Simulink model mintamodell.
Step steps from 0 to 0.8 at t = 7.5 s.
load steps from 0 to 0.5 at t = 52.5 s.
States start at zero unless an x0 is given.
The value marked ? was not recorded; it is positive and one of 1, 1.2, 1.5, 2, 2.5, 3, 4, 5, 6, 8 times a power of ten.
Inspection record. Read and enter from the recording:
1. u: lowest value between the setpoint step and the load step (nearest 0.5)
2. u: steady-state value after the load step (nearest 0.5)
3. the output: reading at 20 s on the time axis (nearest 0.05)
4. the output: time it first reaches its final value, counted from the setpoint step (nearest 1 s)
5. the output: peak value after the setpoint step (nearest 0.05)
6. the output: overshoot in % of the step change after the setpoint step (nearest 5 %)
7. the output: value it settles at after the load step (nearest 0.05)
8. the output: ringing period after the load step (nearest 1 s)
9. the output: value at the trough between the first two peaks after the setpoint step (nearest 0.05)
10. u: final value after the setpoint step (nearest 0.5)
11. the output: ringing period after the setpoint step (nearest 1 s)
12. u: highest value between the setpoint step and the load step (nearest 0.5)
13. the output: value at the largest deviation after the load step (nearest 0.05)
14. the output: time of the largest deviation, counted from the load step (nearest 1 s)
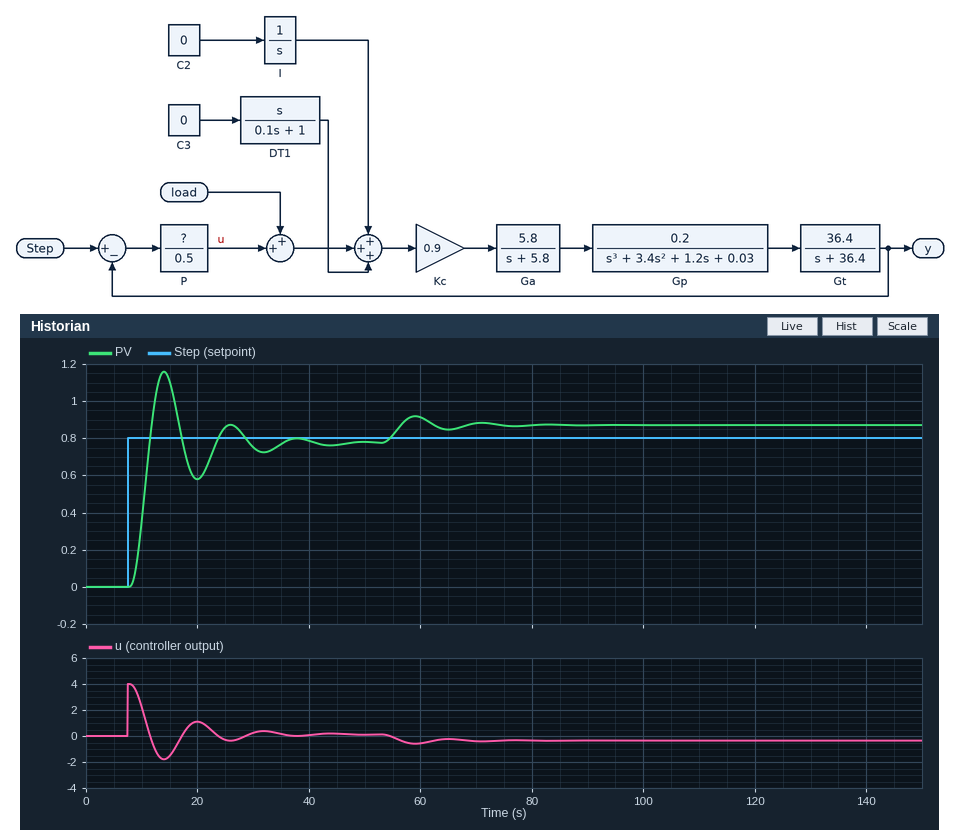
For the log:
-2.0
-0.5
0.60
4 s
1.15
50 %
0.85
12 s
0.60
0.0
12 s
4.0
0.90
7 s
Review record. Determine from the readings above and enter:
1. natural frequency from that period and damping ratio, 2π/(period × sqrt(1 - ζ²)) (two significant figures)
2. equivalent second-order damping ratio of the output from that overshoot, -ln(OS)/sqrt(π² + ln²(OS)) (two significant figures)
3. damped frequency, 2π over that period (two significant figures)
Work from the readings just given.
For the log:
0.54 rad/s
0.22
0.52 rad/s
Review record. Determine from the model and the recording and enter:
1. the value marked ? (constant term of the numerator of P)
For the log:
2.5
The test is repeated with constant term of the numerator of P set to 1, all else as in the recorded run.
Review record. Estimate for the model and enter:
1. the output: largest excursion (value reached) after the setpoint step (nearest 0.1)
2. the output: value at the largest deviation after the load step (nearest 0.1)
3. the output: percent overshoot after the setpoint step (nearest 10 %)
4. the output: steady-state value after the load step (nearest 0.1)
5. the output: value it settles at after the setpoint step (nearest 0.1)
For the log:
0.9
1.0
20 %
1.0
0.7
